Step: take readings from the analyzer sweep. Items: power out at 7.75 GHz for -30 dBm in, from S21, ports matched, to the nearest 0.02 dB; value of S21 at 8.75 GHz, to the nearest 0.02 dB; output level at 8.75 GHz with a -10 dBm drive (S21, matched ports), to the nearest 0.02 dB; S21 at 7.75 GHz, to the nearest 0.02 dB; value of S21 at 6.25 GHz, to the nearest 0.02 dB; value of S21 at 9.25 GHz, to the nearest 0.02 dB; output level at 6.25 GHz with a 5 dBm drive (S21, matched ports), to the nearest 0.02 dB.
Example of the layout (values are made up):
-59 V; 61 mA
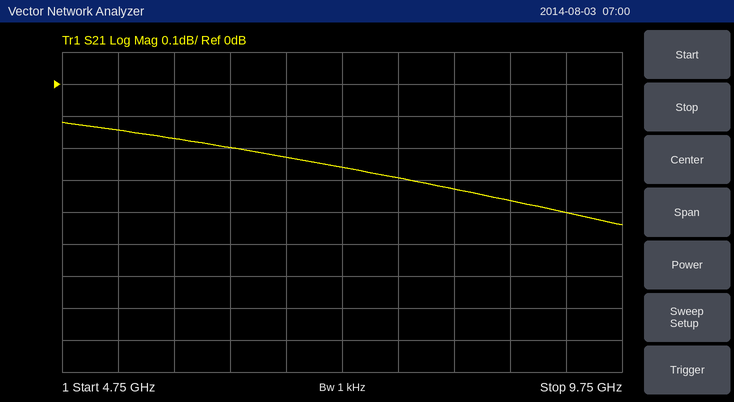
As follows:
-30.30 dBm; -0.36 dB; -10.36 dBm; -0.30 dB; -0.20 dB; -0.40 dB; 4.80 dBm
